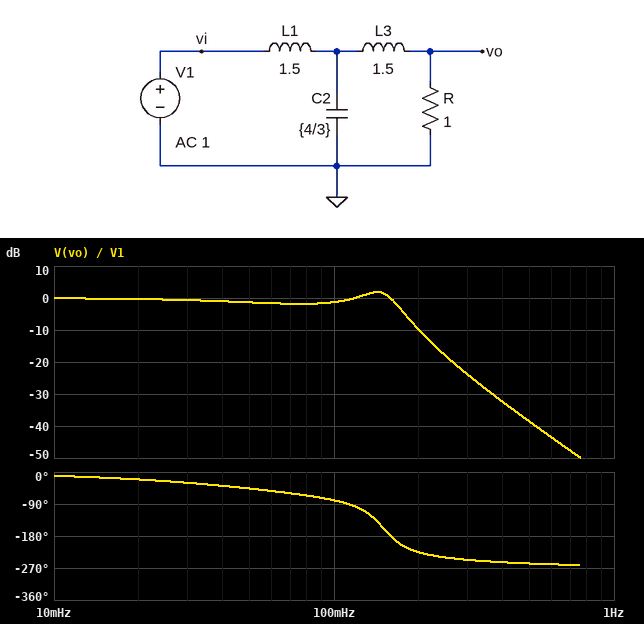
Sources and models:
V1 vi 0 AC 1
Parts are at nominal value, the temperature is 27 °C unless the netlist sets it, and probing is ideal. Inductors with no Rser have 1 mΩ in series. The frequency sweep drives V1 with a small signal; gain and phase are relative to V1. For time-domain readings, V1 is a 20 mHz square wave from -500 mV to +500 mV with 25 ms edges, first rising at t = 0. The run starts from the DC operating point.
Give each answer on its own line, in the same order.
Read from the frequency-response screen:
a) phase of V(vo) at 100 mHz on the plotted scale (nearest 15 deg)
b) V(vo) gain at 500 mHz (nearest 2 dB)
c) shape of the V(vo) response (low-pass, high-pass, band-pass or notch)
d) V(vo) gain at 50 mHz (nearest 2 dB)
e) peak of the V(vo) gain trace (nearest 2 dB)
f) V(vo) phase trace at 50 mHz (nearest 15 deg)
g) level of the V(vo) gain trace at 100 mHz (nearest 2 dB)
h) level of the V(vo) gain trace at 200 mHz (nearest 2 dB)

-75 deg
-38 dB
low-pass
-2 dB
2 dB
-45 deg
-2 dB
-10 dB
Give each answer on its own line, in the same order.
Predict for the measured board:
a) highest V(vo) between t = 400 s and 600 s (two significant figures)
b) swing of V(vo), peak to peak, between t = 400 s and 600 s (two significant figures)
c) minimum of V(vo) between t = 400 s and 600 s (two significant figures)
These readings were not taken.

560 mV
1.1 V
-560 mV
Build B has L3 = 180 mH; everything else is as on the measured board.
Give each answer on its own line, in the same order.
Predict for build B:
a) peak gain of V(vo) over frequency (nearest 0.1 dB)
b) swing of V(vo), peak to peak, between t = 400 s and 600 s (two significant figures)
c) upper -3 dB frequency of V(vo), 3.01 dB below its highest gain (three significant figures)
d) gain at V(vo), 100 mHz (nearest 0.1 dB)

0.6 dB
1.2 V
138 mHz
0.1 dB
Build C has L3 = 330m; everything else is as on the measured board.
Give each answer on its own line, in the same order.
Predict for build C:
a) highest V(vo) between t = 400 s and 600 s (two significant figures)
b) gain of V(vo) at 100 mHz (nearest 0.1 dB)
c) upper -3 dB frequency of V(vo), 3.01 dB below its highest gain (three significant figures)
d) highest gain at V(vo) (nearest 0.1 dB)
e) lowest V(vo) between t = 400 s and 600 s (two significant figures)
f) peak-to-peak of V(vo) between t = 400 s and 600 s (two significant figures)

600 mV
-0.1 dB
147 mHz
0.3 dB
-600 mV
1.2 V
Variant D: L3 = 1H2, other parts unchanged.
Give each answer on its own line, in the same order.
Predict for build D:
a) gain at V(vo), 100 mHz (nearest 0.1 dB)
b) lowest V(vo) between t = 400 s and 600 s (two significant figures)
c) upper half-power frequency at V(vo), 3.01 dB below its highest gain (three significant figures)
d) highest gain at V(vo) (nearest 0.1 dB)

-1.0 dB
-560 mV
171 mHz
0.7 dB
